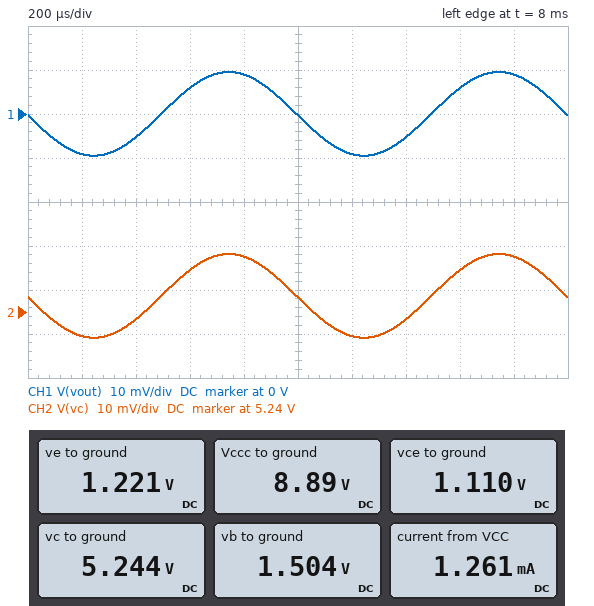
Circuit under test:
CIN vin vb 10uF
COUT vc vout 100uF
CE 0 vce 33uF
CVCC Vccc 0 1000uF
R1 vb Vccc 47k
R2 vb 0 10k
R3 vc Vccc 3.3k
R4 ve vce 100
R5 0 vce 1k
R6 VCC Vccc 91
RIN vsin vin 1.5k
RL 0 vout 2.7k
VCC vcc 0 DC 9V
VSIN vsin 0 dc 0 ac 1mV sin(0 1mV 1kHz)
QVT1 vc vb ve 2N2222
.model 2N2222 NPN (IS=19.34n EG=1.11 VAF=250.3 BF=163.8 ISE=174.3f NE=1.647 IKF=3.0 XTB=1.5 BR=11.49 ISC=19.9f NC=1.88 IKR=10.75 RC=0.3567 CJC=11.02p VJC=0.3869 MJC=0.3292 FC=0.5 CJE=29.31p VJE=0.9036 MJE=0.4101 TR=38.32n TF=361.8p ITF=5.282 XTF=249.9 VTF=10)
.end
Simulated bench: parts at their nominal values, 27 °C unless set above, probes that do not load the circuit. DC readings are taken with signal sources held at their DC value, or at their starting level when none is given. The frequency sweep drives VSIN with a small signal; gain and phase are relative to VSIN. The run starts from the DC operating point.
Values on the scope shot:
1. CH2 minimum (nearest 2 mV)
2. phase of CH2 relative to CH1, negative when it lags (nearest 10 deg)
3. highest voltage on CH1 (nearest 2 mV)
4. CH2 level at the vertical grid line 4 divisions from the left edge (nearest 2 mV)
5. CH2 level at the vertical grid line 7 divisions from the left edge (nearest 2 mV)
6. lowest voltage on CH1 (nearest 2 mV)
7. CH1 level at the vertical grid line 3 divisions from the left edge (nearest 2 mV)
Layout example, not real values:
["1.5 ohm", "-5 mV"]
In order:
["5.234 V", "0 deg", "10 mV", "5.252 V", "5.238 V", "-10 mV", "6 mV"]
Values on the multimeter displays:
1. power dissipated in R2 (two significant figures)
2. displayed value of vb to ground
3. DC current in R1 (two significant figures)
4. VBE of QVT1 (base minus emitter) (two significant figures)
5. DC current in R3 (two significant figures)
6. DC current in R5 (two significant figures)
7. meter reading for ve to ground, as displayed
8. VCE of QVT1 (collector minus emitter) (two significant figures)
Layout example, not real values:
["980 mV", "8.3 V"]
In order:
["230 µW", "1.504 V", "160 µA", "280 mV", "1.1 mA", "1.1 mA", "1.221 V", "4.0 V"]
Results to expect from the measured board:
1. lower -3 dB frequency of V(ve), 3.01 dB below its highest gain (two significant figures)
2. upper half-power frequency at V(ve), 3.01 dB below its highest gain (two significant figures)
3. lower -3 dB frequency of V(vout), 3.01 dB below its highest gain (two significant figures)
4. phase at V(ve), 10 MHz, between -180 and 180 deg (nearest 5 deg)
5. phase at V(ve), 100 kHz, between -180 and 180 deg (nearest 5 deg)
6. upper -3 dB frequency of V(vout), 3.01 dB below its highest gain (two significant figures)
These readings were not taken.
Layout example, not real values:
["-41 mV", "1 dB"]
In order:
["1.6 Hz", "930 kHz", "42 Hz", "-55 deg", "-5 deg", "1.6 MHz"]
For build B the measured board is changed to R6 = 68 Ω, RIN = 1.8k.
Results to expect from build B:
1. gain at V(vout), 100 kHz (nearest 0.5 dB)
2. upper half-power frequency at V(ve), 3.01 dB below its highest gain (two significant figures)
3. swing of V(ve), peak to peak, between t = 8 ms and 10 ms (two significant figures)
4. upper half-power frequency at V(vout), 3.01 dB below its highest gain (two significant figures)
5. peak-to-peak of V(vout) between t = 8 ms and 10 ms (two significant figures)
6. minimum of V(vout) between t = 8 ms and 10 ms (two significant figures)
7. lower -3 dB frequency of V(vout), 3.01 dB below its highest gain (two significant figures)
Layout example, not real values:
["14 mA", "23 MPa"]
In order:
["19.0 dB", "790 kHz", "1.2 mV", "1.4 MHz", "18 mV", "-9.1 mV", "41 Hz"]
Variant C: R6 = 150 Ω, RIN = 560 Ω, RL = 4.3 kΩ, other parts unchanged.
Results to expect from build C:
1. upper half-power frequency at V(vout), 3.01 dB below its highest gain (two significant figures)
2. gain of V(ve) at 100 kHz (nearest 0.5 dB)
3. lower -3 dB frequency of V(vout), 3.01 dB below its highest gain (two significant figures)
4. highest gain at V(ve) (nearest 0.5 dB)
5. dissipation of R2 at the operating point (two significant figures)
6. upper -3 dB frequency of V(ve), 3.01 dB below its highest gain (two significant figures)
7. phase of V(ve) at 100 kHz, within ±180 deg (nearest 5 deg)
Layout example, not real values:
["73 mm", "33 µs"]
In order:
["2.9 MHz", "-2.5 dB", "43 Hz", "-1.0 dB", "220 µW", "1.9 MHz", "0 deg"]
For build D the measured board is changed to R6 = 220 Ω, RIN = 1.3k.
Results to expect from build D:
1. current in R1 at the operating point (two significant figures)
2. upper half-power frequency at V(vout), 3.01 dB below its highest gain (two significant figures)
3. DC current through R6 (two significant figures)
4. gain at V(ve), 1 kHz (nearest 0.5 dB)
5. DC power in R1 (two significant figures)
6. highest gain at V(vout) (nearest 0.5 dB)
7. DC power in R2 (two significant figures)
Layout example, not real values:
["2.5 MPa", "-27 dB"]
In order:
["150 µA", "1.8 MHz", "1.2 mA", "-3.5 dB", "1.1 mW", "20.0 dB", "220 µW"]
